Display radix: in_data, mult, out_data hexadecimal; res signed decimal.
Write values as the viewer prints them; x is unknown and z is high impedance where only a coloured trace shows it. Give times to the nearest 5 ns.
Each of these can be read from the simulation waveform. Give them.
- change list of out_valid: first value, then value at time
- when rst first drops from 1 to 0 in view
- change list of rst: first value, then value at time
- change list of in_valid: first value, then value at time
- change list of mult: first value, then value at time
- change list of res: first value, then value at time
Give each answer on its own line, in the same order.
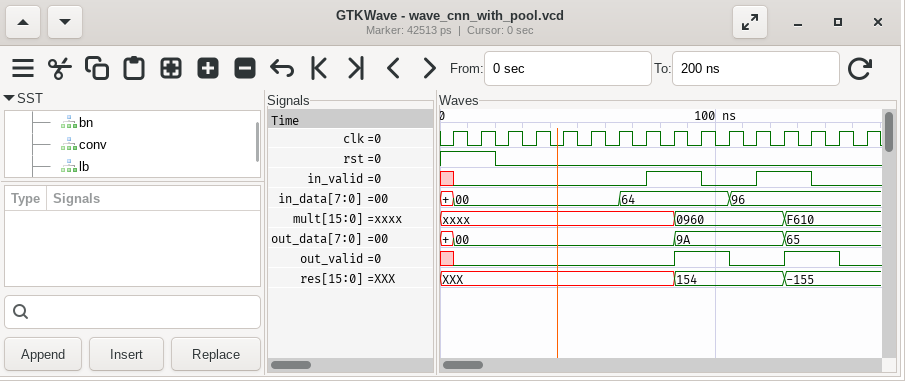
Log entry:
x, 0 at 5 ns, 1 at 85 ns, 0 at 105 ns, 1 at 125 ns, 0 at 145 ns
20 ns
1, 0 at 20 ns
x, 0 at 5 ns, 1 at 75 ns, 0 at 95 ns, 1 at 115 ns, 0 at 135 ns
xxxx, 0960 at 85 ns, F610 at 125 ns
XXX, 154 at 85 ns, -155 at 125 ns
